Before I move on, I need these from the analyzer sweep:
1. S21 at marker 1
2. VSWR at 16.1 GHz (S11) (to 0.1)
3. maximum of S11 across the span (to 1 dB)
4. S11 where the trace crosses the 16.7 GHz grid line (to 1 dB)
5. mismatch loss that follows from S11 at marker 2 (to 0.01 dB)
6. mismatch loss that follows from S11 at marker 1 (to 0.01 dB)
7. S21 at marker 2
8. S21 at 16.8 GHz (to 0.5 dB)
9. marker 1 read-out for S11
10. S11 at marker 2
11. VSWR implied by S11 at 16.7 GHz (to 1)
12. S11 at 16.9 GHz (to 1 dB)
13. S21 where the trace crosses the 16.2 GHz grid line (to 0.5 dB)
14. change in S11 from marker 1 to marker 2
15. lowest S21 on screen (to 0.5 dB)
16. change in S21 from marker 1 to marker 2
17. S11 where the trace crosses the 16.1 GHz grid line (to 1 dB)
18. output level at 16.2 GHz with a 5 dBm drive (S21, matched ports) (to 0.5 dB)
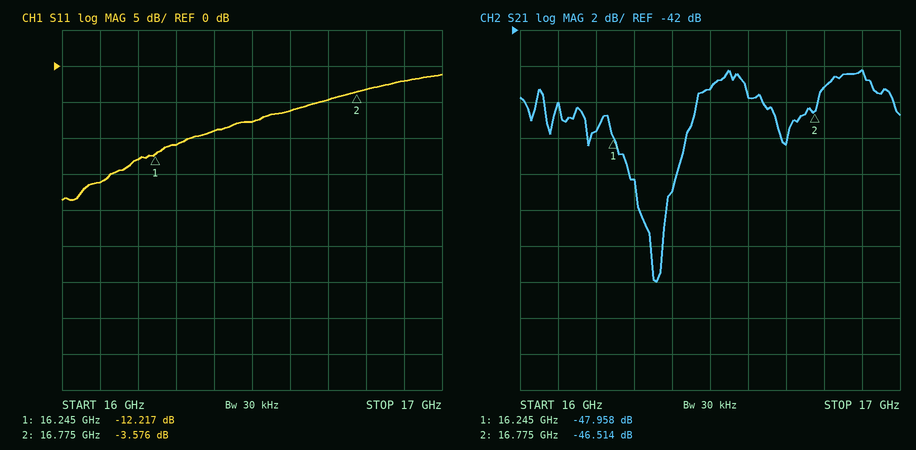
-47.958 dB
1.4
-1 dB
-5 dB
2.51 dB
0.27 dB
-46.514 dB
-45.0 dB
-12.217 dB
-3.576 dB
4
-2 dB
-47.5 dB
8.641 dB
-56.0 dB
1.444 dB
-16 dB
-42.5 dBm
